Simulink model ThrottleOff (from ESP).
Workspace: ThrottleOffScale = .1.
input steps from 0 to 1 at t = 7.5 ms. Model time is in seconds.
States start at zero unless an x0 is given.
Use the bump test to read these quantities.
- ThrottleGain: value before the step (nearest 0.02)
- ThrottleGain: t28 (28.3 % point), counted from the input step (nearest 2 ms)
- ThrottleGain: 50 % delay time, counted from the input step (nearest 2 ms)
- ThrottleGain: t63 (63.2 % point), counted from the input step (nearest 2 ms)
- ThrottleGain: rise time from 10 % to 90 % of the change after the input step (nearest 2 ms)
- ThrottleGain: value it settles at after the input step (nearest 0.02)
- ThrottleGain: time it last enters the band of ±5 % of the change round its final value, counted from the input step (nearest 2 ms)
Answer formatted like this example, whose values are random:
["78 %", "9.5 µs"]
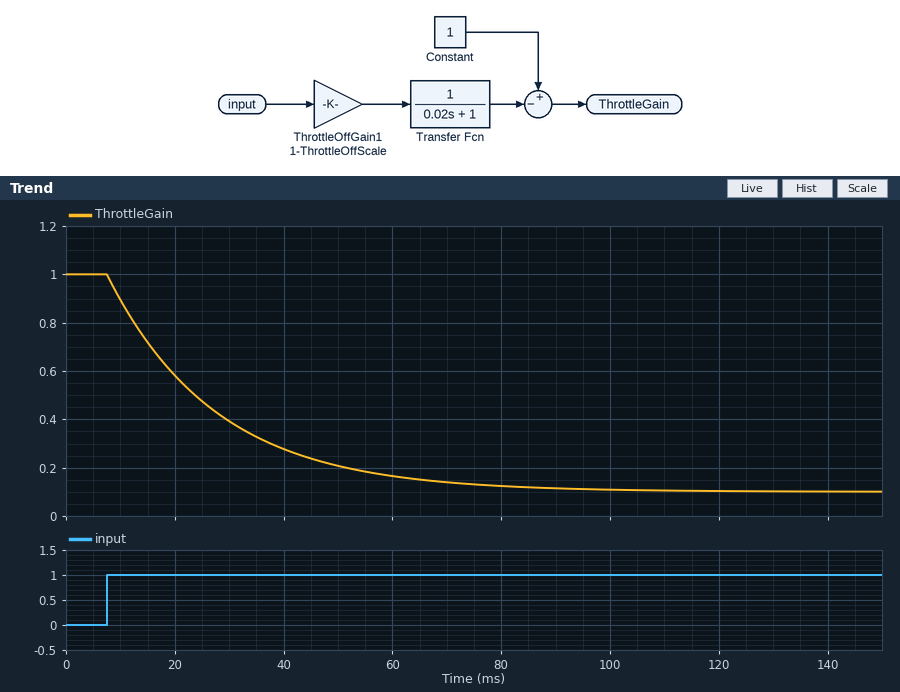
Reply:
["1.00", "6 ms", "14 ms", "20 ms", "44 ms", "0.10", "60 ms"]
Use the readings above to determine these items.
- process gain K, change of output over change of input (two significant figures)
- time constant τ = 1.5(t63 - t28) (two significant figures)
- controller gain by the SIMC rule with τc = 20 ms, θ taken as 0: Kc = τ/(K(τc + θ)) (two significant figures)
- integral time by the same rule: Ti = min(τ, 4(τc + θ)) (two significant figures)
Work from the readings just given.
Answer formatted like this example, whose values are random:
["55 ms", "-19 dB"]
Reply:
["-0.90", "21 ms", "-1.2", "21 ms"]
